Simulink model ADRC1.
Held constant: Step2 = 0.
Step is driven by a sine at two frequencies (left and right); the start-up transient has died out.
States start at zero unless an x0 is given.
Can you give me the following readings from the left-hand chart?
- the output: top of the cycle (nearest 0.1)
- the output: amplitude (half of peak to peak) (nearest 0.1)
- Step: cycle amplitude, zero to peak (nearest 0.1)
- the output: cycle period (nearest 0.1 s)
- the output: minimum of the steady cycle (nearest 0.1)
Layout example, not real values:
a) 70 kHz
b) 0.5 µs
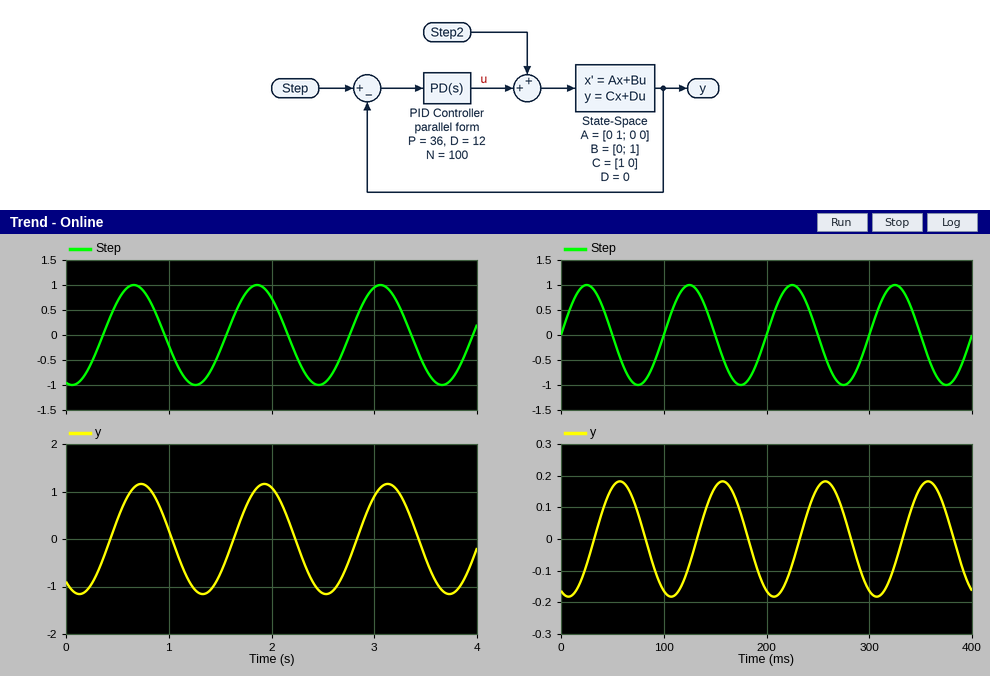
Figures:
a) 1.2
b) 1.2
c) 1.0
d) 1.2 s
e) -1.2
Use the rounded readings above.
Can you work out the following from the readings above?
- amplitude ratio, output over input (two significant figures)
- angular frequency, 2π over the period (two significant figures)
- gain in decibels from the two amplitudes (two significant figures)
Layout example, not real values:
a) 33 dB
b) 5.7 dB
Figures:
a) 1.2
b) 5.2 rad/s
c) 1.6 dB
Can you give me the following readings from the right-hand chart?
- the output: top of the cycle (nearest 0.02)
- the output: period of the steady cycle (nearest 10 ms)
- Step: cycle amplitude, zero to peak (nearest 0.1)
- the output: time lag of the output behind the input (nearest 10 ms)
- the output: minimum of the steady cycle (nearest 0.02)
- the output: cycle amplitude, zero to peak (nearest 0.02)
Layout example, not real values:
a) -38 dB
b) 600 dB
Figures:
a) 0.18
b) 100 ms
c) 1.0
d) 30 ms
e) -0.18
f) 0.18
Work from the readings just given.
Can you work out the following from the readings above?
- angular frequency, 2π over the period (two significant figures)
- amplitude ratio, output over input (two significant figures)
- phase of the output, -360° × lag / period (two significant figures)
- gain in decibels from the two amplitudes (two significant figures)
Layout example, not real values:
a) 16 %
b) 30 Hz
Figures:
a) 0.063 rad/ms
b) 0.18
c) -110°
d) -15 dB
